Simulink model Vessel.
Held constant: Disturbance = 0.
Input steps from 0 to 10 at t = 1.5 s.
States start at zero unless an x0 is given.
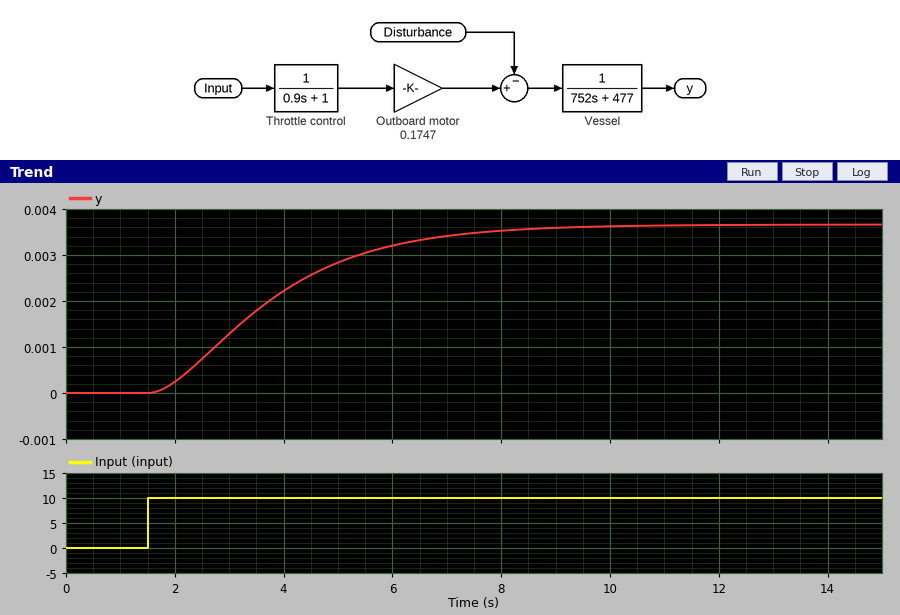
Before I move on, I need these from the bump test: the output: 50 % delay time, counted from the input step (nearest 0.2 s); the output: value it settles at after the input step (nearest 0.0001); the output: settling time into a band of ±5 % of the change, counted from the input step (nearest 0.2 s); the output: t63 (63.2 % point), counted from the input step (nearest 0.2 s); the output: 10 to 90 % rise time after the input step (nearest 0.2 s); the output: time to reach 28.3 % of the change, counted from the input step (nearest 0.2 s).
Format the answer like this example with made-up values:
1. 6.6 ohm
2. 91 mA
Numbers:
1. 2.0 s
2. 0.0037
3. 6.0 s
4. 2.6 s
5. 4.2 s
6. 1.2 s
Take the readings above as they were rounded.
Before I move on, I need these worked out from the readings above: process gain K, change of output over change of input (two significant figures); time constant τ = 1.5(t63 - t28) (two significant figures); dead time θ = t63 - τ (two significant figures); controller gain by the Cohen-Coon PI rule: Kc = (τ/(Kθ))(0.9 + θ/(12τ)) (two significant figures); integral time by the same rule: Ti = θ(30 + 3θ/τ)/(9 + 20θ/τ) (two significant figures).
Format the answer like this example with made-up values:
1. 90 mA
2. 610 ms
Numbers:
1. 0.00037
2. 2.1 s
3. 0.50 s
4. 10000
5. 1.1 s
